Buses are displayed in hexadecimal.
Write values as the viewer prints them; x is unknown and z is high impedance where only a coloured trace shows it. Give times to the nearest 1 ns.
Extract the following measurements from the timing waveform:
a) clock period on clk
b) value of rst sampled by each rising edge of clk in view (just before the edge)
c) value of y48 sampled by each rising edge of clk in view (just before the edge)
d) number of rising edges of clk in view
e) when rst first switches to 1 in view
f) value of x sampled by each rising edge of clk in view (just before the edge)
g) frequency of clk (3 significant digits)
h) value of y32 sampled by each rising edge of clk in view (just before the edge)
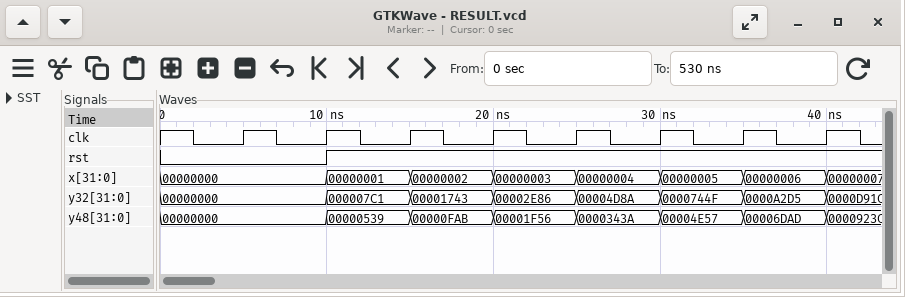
5 ns
0 0 1 1 1 1 1 1
00000000, 00000000, 00000539, 00000FAB, 00001F56, 0000343A, 00004E57, 00006DAD
8
10 ns
00000000, 00000000, 00000001, 00000002, 00000003, 00000004, 00000005, 00000006
200 MHz
00000000, 00000000, 000007C1, 00001743, 00002E86, 00004D8A, 0000744F, 0000A2D5
